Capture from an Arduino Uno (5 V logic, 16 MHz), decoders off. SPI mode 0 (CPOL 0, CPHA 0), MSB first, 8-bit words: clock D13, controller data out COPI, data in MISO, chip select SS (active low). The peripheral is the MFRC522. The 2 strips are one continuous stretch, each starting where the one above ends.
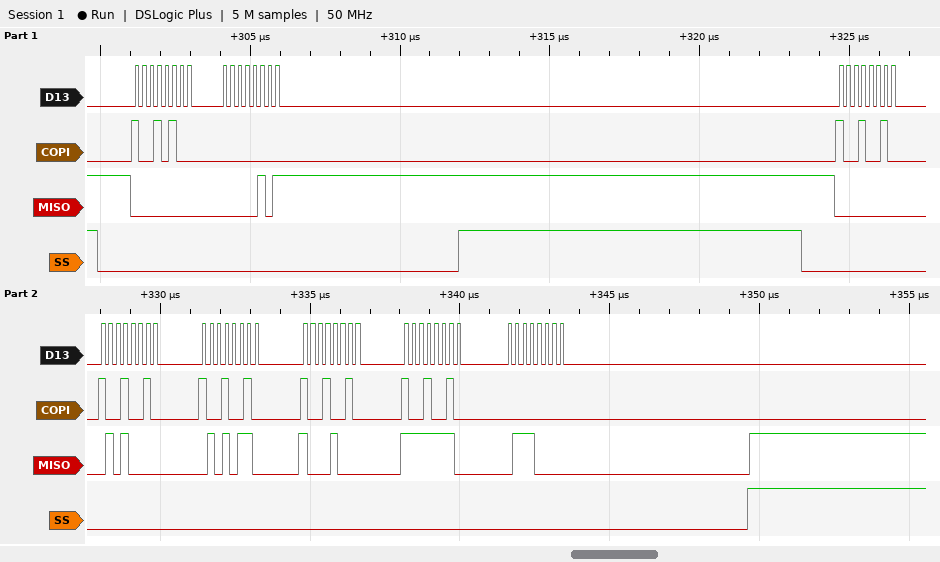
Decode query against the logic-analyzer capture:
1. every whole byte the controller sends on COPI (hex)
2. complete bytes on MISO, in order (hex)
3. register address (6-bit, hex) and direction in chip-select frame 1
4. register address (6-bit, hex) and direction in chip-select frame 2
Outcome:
0x94 0x00 0x92 0x92 0x92 0x92 0x92 0x00
0x00 0x05 0x00 0x50 0x56 0x88 0xFE 0x70
0x0A read
0x09 read
